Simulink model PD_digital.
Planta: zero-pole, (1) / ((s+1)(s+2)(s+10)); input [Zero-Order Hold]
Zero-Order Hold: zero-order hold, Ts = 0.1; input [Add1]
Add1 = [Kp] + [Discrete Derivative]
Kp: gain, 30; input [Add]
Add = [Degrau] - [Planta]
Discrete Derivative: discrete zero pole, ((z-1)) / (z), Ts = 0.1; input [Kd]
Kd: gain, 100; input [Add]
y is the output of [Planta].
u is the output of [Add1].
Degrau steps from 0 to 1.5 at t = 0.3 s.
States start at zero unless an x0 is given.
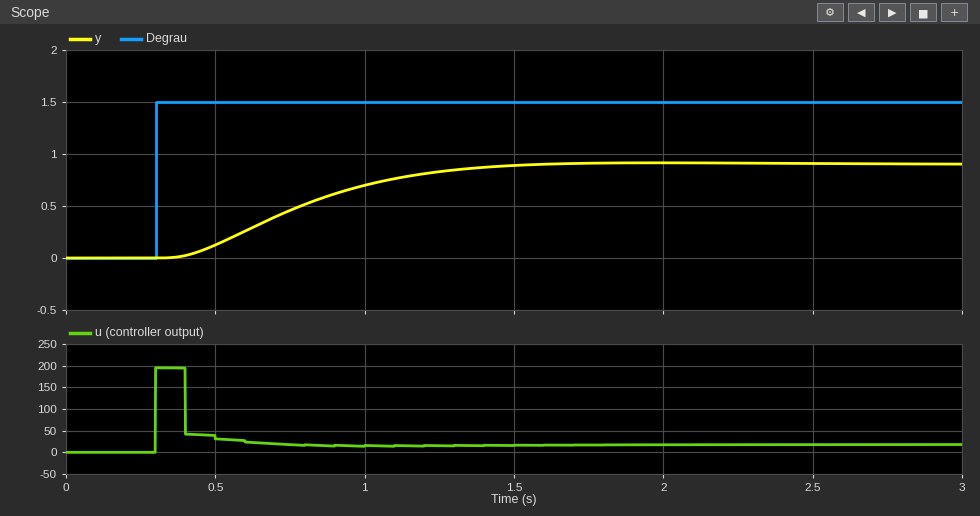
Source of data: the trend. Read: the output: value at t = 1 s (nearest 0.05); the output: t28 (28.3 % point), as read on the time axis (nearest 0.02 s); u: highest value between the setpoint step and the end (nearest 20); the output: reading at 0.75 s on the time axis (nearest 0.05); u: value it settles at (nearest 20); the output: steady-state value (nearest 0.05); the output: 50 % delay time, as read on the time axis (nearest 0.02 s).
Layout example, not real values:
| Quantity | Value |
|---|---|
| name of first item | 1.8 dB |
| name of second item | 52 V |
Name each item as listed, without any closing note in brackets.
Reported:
| Quantity | Value |
|---|---|
| the output: value at t = 1 s | 0.70 |
| the output: t28 (28.3 % point), as read on the time axis | 0.60 s |
| u: highest value between the setpoint step and the end | 200 |
| the output: reading at 0.75 s on the time axis | 0.45 |
| u: value it settles at | 20 |
| the output: steady-state value | 0.90 |
| the output: 50 % delay time, as read on the time axis | 0.74 s |
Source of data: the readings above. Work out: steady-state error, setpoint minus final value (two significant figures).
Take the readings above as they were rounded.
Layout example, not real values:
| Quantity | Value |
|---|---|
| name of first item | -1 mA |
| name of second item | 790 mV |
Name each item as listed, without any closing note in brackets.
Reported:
| Quantity | Value |
|---|---|
| steady-state error, setpoint minus final value | 0.60 |
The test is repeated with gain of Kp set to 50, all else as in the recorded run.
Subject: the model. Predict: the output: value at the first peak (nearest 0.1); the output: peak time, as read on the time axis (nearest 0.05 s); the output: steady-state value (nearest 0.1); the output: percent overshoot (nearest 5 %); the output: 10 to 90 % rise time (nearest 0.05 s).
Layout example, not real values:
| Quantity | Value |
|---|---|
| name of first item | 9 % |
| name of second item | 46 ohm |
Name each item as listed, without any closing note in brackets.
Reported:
| Quantity | Value |
|---|---|
| the output: value at the first peak | 1.2 |
| the output: peak time, as read on the time axis | 1.55 s |
| the output: steady-state value | 1.1 |
| the output: percent overshoot | 10 % |
| the output: 10 to 90 % rise time | 0.55 s |
